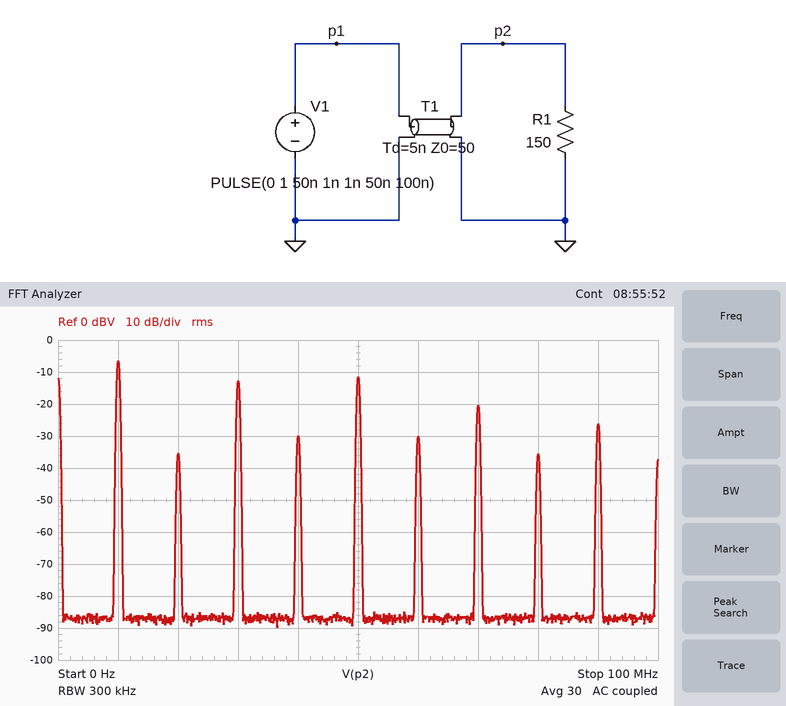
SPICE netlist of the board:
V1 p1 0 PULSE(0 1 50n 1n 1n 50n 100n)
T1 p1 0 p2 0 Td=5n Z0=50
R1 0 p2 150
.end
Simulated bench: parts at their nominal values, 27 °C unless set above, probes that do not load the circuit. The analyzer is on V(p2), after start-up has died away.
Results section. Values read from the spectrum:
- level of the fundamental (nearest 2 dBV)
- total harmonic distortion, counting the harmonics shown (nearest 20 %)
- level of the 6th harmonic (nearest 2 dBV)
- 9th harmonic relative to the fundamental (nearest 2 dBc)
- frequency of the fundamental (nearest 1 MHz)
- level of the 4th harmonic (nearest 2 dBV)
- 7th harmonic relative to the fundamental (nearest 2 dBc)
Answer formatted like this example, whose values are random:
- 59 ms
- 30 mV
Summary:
- -6 dBV
- 80 %
- -30 dBV
- -20 dBc
- 10 MHz
- -30 dBV
- -14 dBc
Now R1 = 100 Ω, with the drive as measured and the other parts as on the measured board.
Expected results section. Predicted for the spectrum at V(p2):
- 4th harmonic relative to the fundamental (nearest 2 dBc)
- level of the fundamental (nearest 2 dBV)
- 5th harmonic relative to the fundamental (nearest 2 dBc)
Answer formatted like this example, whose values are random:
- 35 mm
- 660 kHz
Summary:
- -26 dBc
- -6 dBV
- -8 dBc
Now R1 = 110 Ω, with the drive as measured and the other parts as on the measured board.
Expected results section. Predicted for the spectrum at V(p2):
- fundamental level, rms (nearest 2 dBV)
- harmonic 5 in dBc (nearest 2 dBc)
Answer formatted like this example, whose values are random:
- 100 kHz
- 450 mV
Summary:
- -6 dBV
- -8 dBc
